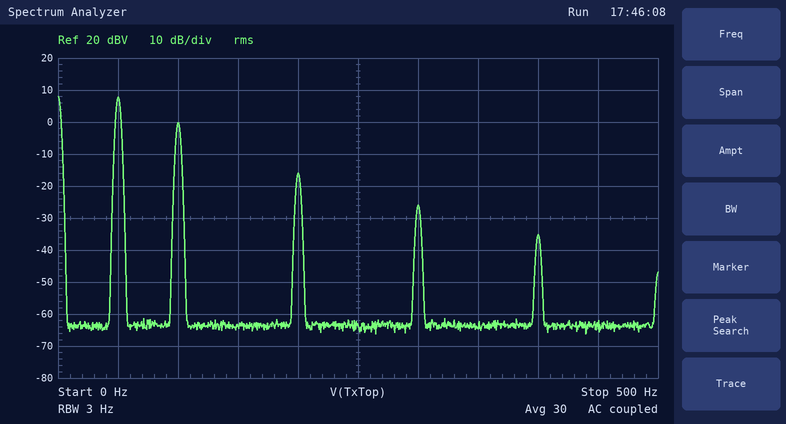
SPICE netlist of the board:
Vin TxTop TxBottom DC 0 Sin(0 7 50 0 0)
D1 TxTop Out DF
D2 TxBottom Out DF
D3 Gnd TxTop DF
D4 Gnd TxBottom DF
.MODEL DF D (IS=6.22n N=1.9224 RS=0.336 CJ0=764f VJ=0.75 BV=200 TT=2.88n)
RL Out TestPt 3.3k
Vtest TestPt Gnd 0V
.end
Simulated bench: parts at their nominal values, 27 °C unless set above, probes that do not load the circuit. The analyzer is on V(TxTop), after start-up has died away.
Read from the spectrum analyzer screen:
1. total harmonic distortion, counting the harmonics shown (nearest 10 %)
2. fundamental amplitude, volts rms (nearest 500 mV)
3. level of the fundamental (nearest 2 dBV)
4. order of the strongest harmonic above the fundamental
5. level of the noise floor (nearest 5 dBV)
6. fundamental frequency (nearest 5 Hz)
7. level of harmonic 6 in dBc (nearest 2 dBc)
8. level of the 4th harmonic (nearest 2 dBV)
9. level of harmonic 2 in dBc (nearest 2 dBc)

40 %
2.5 V
8 dBV
2
-65 dBV
50 Hz
-34 dBc
-16 dBV
-8 dBc
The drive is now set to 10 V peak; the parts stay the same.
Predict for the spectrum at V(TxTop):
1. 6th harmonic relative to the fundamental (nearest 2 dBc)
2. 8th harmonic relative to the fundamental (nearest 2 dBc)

-32 dBc
-38 dBc
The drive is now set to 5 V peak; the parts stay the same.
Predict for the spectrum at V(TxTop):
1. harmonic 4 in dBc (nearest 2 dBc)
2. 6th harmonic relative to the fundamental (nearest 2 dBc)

-26 dBc
-38 dBc
